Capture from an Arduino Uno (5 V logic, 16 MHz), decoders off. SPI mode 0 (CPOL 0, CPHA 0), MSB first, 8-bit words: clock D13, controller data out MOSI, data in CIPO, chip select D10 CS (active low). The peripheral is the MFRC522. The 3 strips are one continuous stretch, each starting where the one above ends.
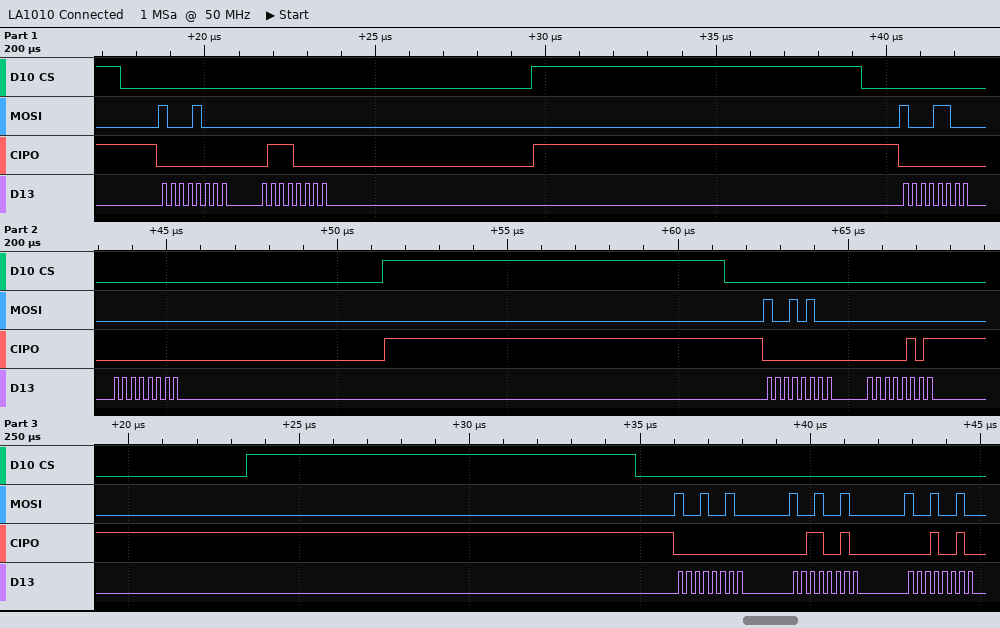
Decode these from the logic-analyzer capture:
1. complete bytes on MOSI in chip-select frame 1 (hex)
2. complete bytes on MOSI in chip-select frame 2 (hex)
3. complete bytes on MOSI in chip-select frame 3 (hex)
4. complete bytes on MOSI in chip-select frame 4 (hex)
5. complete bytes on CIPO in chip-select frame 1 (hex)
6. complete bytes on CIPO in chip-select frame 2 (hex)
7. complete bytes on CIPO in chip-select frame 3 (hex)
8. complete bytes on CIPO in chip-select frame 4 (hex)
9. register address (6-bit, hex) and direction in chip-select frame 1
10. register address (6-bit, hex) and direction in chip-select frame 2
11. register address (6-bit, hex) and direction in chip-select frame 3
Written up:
88 00
8C 00
94 00
92 92 92
00 70
00 00
00 05
00 32 12
0x04 read
0x06 read
0x0A read
